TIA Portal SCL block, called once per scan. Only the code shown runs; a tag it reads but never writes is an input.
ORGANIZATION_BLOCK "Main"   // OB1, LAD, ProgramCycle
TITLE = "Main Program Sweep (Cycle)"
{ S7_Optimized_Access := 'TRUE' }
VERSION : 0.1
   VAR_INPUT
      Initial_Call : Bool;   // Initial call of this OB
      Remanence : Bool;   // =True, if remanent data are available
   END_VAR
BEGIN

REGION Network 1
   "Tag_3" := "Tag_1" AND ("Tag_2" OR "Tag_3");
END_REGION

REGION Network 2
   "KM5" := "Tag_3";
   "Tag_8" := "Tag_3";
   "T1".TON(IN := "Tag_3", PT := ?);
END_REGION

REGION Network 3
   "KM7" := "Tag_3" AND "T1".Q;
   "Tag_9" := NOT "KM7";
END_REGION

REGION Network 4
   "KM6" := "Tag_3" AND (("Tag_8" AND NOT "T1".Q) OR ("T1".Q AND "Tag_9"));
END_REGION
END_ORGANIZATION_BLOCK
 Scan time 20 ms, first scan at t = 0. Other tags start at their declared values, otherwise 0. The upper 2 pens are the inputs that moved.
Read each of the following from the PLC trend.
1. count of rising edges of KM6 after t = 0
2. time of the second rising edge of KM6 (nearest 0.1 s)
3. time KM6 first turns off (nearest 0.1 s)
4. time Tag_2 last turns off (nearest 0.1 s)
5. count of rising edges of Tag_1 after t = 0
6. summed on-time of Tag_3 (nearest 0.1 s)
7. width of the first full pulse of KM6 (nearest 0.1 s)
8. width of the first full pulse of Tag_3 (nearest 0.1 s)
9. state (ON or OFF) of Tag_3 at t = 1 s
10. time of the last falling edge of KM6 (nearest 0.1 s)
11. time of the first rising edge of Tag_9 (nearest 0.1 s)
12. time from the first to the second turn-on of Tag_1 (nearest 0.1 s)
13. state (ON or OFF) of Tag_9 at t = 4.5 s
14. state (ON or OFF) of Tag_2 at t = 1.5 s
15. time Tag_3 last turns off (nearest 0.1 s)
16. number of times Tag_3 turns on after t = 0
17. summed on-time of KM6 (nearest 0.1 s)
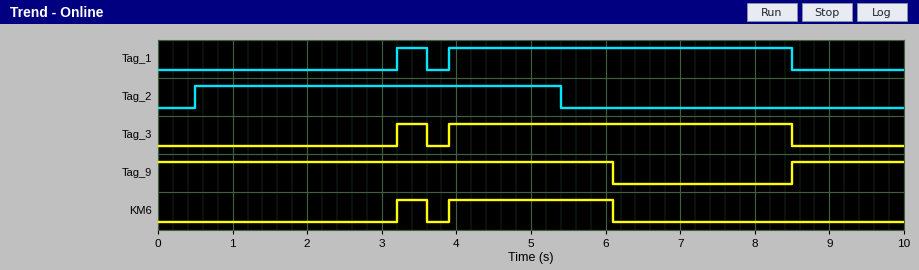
2
3.9 s
3.6 s
5.4 s
2
5.0 s
0.4 s
0.4 s
OFF
6.1 s
8.5 s
0.7 s
ON
ON
8.5 s
2
2.6 s
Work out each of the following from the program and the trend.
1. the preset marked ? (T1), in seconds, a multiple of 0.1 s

2.2 s
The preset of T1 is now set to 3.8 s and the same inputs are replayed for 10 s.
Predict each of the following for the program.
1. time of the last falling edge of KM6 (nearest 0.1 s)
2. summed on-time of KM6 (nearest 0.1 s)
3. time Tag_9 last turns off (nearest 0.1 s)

7.7 s
4.2 s
7.7 s
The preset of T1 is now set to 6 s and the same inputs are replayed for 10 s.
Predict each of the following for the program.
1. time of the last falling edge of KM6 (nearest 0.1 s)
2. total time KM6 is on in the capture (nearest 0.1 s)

8.5 s
5.0 s
